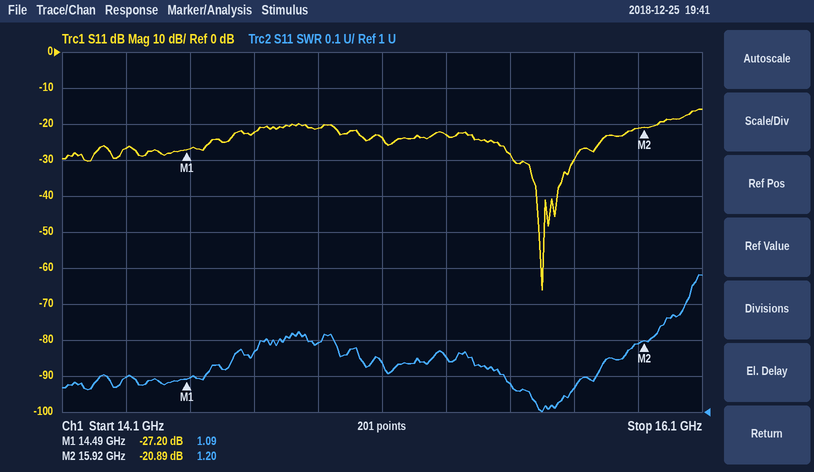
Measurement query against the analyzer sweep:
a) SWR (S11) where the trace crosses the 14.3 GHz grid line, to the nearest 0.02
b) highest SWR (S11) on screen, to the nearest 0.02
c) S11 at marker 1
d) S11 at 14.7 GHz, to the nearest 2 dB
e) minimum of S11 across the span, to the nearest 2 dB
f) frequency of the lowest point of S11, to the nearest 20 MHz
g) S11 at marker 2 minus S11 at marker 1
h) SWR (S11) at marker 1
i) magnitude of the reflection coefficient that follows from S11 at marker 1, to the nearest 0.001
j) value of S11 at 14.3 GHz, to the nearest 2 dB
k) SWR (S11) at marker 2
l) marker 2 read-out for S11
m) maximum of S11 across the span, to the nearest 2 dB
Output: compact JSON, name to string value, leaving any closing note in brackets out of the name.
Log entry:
{"SWR (S11) where the trace crosses the 14.3 GHz grid line, to the nearest 0.02": "1.10", "highest SWR (S11) on screen, to the nearest 0.02": "1.38", "S11 at marker 1": "-27.20 dB", "S11 at 14.7 GHz, to the nearest 2 dB": "-22 dB", "minimum of S11 across the span, to the nearest 2 dB": "-66 dB", "frequency of the lowest point of S11, to the nearest 20 MHz": "15.60 GHz", "S11 at marker 2 minus S11 at marker 1": "6.31 dB", "SWR (S11) at marker 1": "1.09", "magnitude of the reflection coefficient that follows from S11 at marker 1, to the nearest 0.001": "0.044", "value of S11 at 14.3 GHz, to the nearest 2 dB": "-26 dB", "SWR (S11) at marker 2": "1.20", "marker 2 read-out for S11": "-20.89 dB", "maximum of S11 across the span, to the nearest 2 dB": "-16 dB"}
